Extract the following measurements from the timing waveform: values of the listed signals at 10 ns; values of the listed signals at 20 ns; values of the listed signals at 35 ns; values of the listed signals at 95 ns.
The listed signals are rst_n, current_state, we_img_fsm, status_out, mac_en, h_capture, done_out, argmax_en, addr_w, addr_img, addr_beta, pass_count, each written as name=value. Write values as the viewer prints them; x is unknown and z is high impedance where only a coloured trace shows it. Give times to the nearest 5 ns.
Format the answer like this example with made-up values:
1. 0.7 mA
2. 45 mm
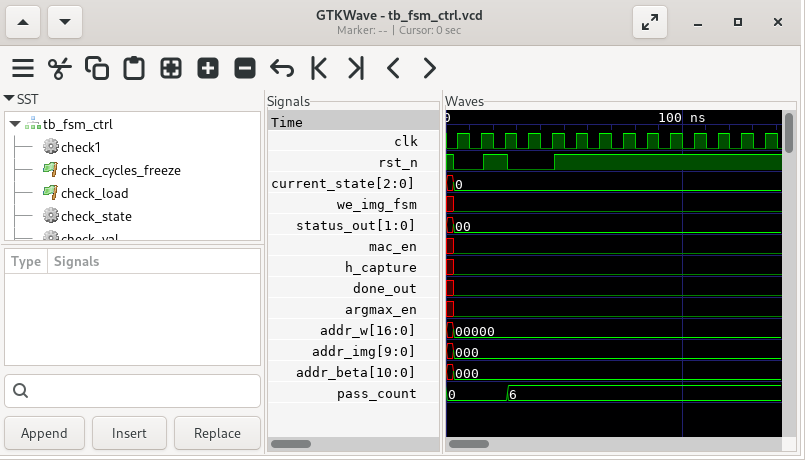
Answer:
1. rst_n=0, current_state=0, we_img_fsm=0, status_out=00, mac_en=0, h_capture=0, done_out=0, argmax_en=0, addr_w=00000, addr_img=000, addr_beta=000, pass_count=0
2. rst_n=1, current_state=0, we_img_fsm=0, status_out=00, mac_en=0, h_capture=0, done_out=0, argmax_en=0, addr_w=00000, addr_img=000, addr_beta=000, pass_count=0
3. rst_n=0, current_state=0, we_img_fsm=0, status_out=00, mac_en=0, h_capture=0, done_out=0, argmax_en=0, addr_w=00000, addr_img=000, addr_beta=000, pass_count=6
4. rst_n=1, current_state=0, we_img_fsm=0, status_out=00, mac_en=0, h_capture=0, done_out=0, argmax_en=0, addr_w=00000, addr_img=000, addr_beta=000, pass_count=6
